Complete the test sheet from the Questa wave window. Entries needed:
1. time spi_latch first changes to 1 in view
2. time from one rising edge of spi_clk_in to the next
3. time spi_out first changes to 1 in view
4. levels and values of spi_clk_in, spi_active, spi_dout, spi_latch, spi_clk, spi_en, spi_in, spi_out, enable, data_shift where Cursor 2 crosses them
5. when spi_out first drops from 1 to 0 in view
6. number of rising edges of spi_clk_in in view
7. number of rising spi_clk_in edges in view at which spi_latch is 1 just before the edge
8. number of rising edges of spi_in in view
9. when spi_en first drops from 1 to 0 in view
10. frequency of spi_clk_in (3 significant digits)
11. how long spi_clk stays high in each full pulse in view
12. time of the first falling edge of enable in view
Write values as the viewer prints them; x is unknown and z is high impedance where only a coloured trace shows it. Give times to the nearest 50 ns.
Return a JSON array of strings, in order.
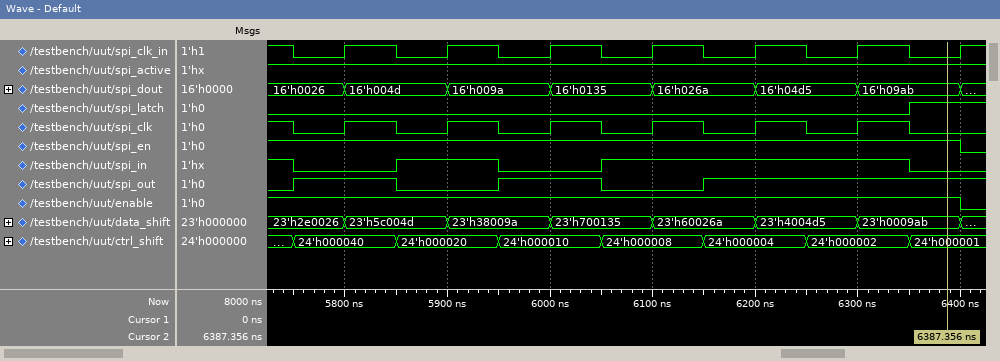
["6350 ns", "100 ns", "5750 ns", "spi_clk_in=0, spi_active=1, spi_dout=16'h09ab, spi_latch=1, spi_clk=0, spi_en=1, spi_in=0, spi_out=1, enable=1, data_shift=23'h0009ab", "5850 ns", "7", "1", "2", "6400 ns", "10.0 MHz", "50 ns, 50 ns, 50 ns, 50 ns, 50 ns, 50 ns", "6400 ns"]
